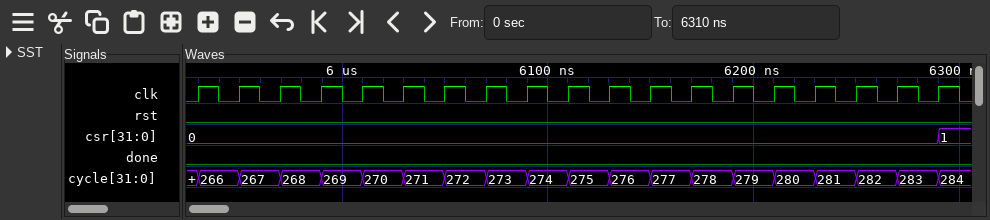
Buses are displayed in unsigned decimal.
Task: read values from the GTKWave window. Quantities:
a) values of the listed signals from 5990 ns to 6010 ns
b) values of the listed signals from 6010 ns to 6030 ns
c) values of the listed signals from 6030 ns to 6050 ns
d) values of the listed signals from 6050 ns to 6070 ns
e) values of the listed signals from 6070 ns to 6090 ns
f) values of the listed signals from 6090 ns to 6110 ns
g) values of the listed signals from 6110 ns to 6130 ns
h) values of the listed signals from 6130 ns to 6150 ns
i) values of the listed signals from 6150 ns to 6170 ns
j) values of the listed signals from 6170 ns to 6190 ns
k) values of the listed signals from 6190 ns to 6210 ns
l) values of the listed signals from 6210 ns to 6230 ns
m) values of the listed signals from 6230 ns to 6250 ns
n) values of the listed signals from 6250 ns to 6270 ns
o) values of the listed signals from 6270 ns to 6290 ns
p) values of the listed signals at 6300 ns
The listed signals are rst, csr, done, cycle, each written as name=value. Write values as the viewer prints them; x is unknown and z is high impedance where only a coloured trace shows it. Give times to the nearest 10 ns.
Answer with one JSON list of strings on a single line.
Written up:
["rst=0, csr=0, done=0, cycle=269", "rst=0, csr=0, done=0, cycle=270", "rst=0, csr=0, done=0, cycle=271", "rst=0, csr=0, done=0, cycle=272", "rst=0, csr=0, done=0, cycle=273", "rst=0, csr=0, done=0, cycle=274", "rst=0, csr=0, done=0, cycle=275", "rst=0, csr=0, done=0, cycle=276", "rst=0, csr=0, done=0, cycle=277", "rst=0, csr=0, done=0, cycle=278", "rst=0, csr=0, done=0, cycle=279", "rst=0, csr=0, done=0, cycle=280", "rst=0, csr=0, done=0, cycle=281", "rst=0, csr=0, done=0, cycle=282", "rst=0, csr=0, done=0, cycle=283", "rst=0, csr=1, done=0, cycle=284"]
